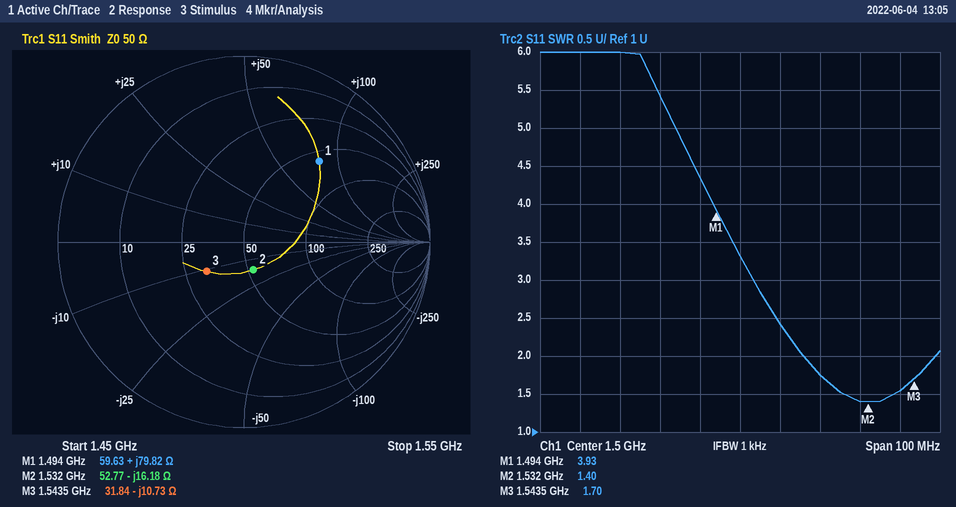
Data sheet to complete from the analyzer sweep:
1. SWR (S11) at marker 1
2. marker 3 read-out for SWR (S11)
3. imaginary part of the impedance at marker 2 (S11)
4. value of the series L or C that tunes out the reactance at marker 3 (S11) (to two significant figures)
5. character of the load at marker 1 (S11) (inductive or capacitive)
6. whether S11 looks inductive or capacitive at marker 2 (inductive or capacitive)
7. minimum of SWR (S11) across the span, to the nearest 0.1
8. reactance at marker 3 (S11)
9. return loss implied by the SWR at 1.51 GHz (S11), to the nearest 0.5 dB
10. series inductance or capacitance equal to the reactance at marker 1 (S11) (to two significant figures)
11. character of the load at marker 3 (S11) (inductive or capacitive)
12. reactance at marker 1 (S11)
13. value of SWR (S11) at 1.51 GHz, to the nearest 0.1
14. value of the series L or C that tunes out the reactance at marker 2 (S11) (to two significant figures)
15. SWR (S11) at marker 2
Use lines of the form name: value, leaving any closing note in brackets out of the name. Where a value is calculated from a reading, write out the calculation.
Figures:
SWR (S11) at marker 1: 3.93
marker 3 read-out for SWR: 1.70
imaginary part of the impedance at marker 2: -16.18 Ω
value of the series L or C that tunes out the reactance at marker 3 (S11): L = 10.73 Ω/(2π × 1.5435 GHz) ≈ 1.1 nH
character of the load at marker 1 (S11): inductive
whether S11 looks inductive or capacitive at marker 2: capacitive
minimum of SWR (S11) across the span, to the nearest 0.1: 1.4
reactance at marker 3: -10.73 Ω
return loss implied by the SWR at 1.51 GHz (S11), to the nearest 0.5 dB: −20 log10((2.4 − 1)/(2.4 + 1)) ≈ 7.71 dB, so 7.5 dB to the nearest 0.5 dB
series inductance or capacitance equal to the reactance at marker 1 (S11): L = 79.82 Ω/(2π × 1.494 GHz) ≈ 8.5 nH
character of the load at marker 3 (S11): capacitive
reactance at marker 1: +79.82 Ω
value of SWR (S11) at 1.51 GHz, to the nearest 0.1: 2.4
value of the series L or C that tunes out the reactance at marker 2 (S11): L = 16.18 Ω/(2π × 1.532 GHz) ≈ 1.7 nH
SWR (S11) at marker 2: 1.40
